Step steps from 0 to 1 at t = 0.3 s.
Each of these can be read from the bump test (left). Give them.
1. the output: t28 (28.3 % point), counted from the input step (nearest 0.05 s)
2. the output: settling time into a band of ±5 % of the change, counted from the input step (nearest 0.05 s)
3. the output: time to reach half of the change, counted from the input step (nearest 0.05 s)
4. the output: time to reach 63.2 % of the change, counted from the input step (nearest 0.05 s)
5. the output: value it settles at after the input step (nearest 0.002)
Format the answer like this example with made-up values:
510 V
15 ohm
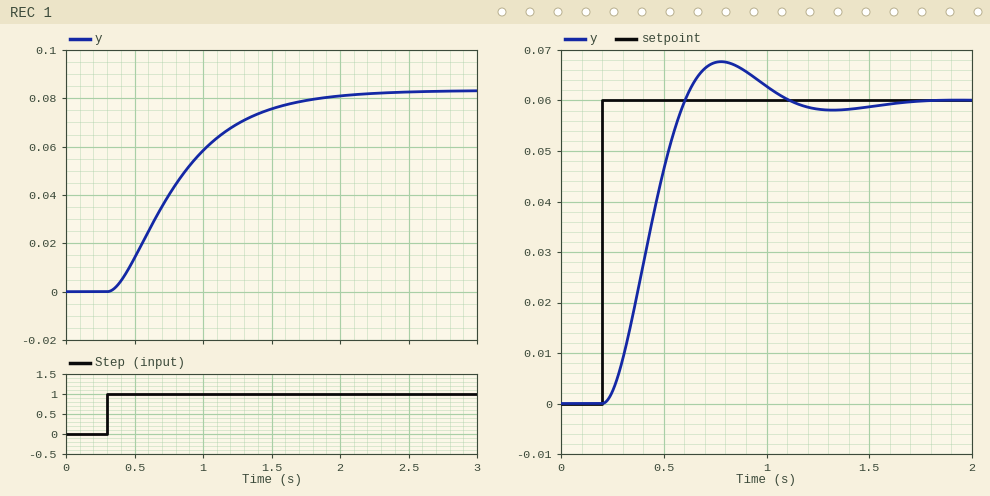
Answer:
0.30 s
1.45 s
0.45 s
0.60 s
0.084
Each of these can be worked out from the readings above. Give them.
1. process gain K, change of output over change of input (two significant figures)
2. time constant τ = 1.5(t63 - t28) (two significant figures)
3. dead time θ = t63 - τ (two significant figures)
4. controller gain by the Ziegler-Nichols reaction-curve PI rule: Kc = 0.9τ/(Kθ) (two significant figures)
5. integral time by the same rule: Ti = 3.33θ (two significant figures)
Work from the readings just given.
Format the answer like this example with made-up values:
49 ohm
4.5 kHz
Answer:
0.084
0.45 s
0.15 s
32
0.50 s
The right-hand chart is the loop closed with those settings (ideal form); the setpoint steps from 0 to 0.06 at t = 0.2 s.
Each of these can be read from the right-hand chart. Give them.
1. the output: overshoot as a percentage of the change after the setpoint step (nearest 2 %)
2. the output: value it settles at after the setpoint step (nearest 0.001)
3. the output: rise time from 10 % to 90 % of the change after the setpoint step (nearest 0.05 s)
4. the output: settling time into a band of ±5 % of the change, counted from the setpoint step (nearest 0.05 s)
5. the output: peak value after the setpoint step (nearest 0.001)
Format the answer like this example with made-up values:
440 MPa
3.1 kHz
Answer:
12 %
0.060
0.25 s
0.80 s
0.068
